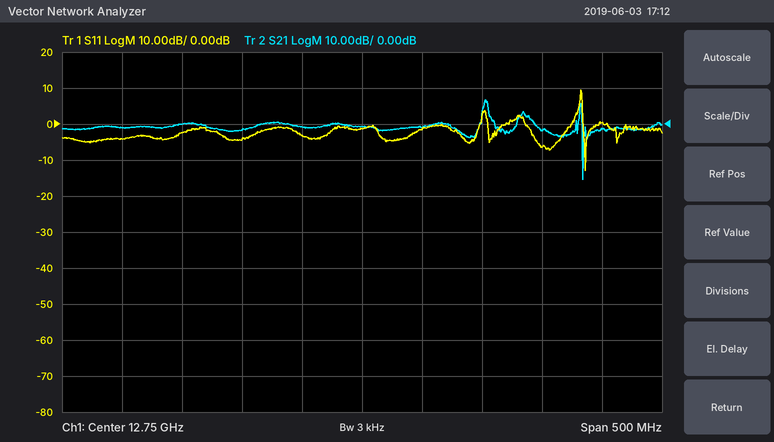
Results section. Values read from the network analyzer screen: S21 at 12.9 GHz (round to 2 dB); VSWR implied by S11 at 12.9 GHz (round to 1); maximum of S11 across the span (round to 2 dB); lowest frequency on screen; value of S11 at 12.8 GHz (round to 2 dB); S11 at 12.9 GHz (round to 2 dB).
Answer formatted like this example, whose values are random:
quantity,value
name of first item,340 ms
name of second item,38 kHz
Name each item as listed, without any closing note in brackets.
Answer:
quantity,value
S21 at 12.9 GHz,-2 dB
VSWR implied by S11 at 12.9 GHz,3
maximum of S11 across the span,10 dB
lowest frequency on screen,12.5 GHz
value of S11 at 12.8 GHz,-2 dB
S11 at 12.9 GHz,-6 dB
